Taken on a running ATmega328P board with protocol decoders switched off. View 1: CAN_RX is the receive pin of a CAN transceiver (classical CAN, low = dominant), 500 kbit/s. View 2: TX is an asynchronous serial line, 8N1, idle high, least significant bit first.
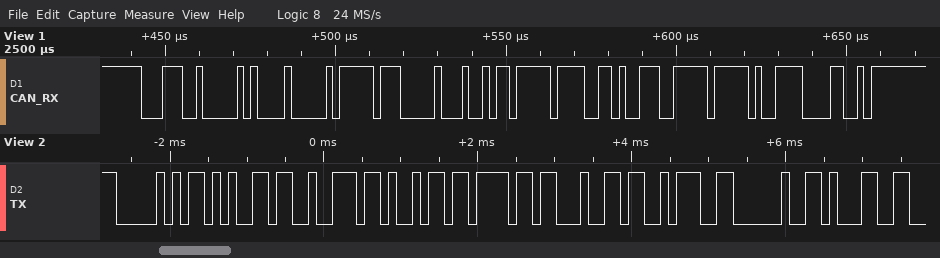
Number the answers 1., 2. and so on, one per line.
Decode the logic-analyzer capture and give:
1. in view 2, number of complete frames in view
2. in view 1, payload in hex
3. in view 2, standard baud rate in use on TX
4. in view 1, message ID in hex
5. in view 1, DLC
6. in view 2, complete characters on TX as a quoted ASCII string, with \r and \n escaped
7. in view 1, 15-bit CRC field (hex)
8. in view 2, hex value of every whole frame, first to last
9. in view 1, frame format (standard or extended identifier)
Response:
1. 9
2. 40 FF 00 96 FF 9A 73 FF
3. 9600 baud
4. 0x1C8
5. 8
6. "Period: 1"
7. 0x4F0C
8. 50 65 72 69 6F 64 3A 20 31
9. standard
